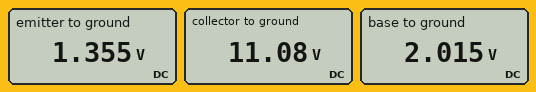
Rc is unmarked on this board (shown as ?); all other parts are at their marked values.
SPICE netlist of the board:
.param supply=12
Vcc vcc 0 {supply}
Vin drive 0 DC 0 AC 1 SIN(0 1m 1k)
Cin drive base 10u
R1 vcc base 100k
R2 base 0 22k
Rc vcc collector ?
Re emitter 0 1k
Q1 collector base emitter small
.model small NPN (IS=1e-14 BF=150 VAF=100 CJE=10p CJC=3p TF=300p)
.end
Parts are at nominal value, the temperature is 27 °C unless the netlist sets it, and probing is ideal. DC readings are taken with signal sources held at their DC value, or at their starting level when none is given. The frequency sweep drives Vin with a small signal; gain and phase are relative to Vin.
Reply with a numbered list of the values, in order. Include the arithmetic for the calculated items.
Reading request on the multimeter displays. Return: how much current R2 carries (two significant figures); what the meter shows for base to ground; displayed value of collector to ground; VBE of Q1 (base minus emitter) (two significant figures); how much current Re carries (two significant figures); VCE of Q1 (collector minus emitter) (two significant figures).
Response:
1. (2.015 V) / 22 kΩ = 92 µA
2. 2.015 V
3. 11.08 V
4. 2.015 V - 1.355 V = 660 mV
5. (1.355 V) / 1 kΩ = 1.4 mA
6. 11.08 V - 1.355 V = 9.7 V
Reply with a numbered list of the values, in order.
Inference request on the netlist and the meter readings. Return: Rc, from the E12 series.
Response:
1. 680 Ω
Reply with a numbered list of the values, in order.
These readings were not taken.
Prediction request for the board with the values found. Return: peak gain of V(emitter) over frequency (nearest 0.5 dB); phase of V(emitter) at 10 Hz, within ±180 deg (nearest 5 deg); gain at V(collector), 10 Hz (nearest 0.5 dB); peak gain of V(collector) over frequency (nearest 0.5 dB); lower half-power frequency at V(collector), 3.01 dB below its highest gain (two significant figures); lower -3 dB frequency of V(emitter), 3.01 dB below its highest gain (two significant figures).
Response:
1. 0 dB
2. 5 deg
3. -3.5 dB
4. -3.5 dB
5. 980 mHz
6. 980 mHz
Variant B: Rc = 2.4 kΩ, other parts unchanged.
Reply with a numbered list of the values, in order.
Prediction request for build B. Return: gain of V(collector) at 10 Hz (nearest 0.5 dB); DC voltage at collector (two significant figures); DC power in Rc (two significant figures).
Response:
1. 7.5 dB
2. 8.8 V
3. 4.3 mW
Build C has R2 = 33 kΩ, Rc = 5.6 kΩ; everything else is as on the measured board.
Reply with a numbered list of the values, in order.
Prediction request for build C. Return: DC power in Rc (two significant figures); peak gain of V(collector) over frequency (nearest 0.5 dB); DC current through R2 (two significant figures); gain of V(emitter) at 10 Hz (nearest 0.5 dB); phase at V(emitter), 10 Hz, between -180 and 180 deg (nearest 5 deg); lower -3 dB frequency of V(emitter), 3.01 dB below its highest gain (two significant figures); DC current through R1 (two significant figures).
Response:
1. 18 mW
2. 3.0 dB
3. 75 µA
4. -4.0 dB
5. 50 deg
6. 12 Hz
7. 95 µA
